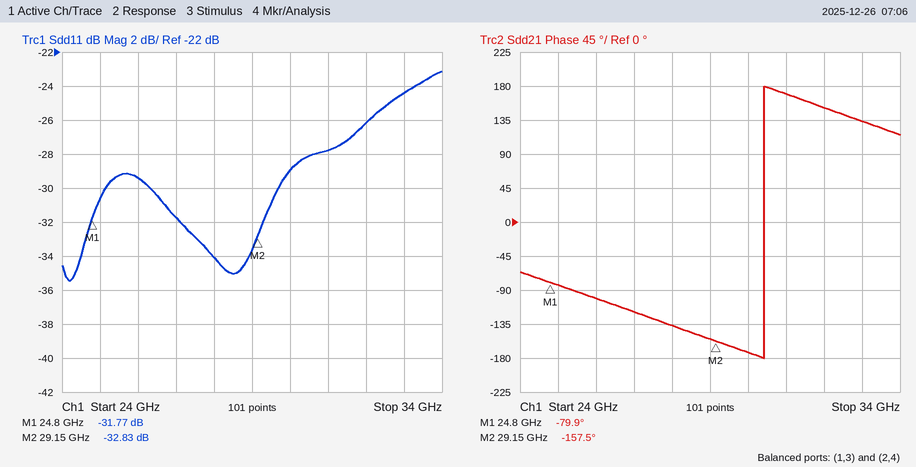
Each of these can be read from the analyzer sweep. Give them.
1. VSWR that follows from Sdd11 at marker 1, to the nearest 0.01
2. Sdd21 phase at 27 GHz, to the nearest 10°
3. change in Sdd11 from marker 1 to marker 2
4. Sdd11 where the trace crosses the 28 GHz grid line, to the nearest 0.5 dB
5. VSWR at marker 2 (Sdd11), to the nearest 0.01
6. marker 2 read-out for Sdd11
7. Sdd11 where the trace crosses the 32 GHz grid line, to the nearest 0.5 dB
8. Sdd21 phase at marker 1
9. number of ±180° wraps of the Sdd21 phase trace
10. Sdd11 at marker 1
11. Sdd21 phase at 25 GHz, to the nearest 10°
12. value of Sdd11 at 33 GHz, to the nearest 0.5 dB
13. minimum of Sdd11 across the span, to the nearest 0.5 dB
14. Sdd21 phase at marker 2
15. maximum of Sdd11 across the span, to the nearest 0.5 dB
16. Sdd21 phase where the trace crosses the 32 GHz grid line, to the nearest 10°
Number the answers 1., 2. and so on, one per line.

1. 1.05
2. -120°
3. -1.06 dB
4. -34.0 dB
5. 1.05
6. -32.83 dB
7. -26.0 dB
8. -79.9°
9. 1
10. -31.77 dB
11. -80°
12. -24.5 dB
13. -35.5 dB
14. -157.5°
15. -23.0 dB
16. 150°
